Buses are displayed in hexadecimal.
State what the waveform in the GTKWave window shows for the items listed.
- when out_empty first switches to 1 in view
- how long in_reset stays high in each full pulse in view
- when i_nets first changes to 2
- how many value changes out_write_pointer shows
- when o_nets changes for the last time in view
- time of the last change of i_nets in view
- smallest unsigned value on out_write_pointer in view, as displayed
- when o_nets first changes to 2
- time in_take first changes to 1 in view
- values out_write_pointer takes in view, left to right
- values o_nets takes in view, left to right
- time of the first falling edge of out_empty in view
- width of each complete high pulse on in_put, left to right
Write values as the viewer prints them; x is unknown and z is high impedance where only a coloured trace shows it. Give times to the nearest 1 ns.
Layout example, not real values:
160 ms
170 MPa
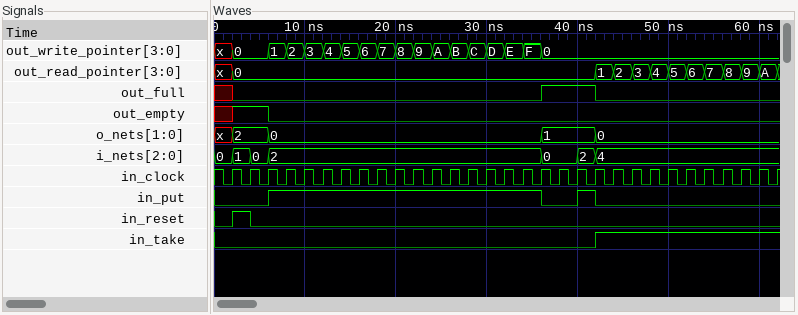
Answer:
2 ns
2 ns
6 ns
17
42 ns
42 ns
0
2 ns
42 ns
x, 0, 1, 2, 3, 4, 5, 6, 7, 8, 9, A, B, C, D, E, F, 0
x, 2, 0, 1, 0
6 ns
30 ns, 2 ns
